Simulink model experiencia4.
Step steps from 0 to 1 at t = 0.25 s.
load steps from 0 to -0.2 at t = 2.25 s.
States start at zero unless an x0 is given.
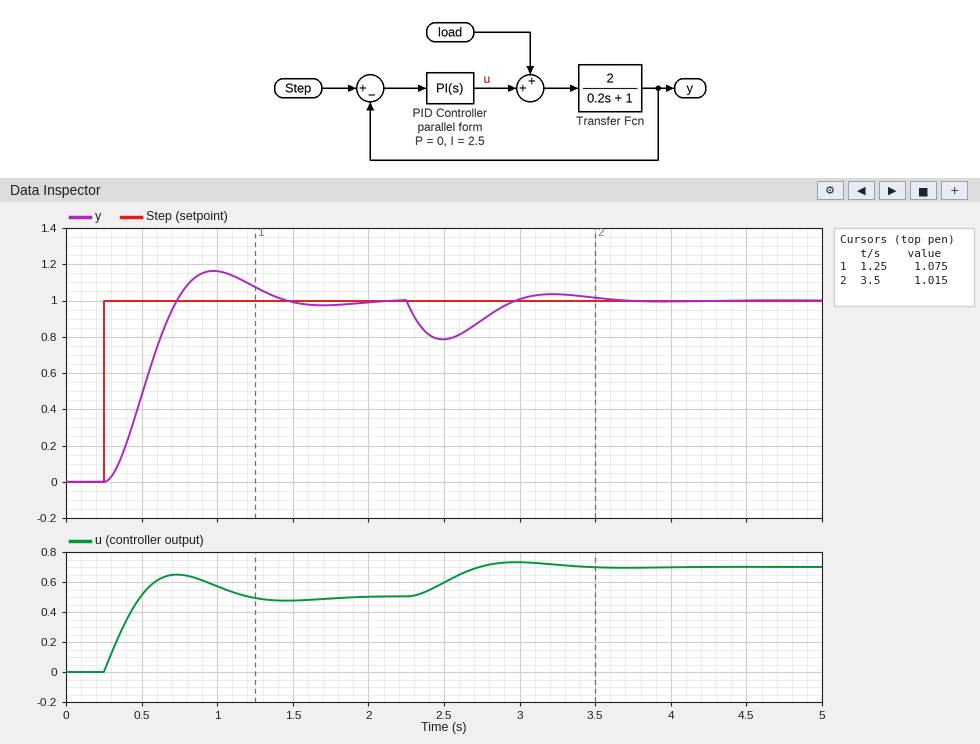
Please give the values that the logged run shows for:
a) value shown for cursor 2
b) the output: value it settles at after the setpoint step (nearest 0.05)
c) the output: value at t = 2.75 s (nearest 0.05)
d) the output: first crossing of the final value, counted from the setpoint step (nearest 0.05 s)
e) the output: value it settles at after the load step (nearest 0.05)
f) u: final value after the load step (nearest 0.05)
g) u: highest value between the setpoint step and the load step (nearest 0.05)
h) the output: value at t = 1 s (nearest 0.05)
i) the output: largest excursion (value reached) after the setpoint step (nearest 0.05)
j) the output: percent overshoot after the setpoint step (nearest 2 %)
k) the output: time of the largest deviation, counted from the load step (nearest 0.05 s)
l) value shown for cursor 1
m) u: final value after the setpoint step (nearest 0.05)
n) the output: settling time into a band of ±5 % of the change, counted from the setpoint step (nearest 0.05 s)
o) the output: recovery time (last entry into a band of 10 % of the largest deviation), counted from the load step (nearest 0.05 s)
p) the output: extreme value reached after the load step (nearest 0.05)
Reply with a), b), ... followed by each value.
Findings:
a) 1.015
b) 1.00
c) 0.90
d) 0.50 s
e) 1.00
f) 0.70
g) 0.65
h) 1.15
i) 1.15
j) 16 %
k) 0.25 s
l) 1.075
m) 0.50
n) 1.05 s
o) 1.20 s
p) 0.80
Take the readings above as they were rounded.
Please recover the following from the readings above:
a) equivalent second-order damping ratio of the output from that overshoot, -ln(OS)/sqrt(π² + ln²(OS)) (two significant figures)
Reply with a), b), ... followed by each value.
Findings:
a) 0.50
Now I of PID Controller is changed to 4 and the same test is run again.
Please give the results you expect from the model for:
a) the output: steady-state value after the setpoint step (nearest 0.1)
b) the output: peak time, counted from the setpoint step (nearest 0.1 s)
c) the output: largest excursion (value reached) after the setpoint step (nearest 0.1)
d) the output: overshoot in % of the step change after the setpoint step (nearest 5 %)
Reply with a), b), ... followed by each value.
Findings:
a) 1.0
b) 0.5 s
c) 1.3
d) 25 %
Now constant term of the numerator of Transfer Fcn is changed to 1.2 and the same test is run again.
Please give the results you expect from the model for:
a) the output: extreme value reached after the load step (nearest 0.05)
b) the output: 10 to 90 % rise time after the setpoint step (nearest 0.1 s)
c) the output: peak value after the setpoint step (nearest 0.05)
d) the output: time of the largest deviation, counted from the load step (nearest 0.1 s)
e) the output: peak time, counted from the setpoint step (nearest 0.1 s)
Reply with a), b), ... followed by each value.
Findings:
a) 0.85
b) 0.5 s
c) 1.05
d) 0.3 s
e) 1.1 s
